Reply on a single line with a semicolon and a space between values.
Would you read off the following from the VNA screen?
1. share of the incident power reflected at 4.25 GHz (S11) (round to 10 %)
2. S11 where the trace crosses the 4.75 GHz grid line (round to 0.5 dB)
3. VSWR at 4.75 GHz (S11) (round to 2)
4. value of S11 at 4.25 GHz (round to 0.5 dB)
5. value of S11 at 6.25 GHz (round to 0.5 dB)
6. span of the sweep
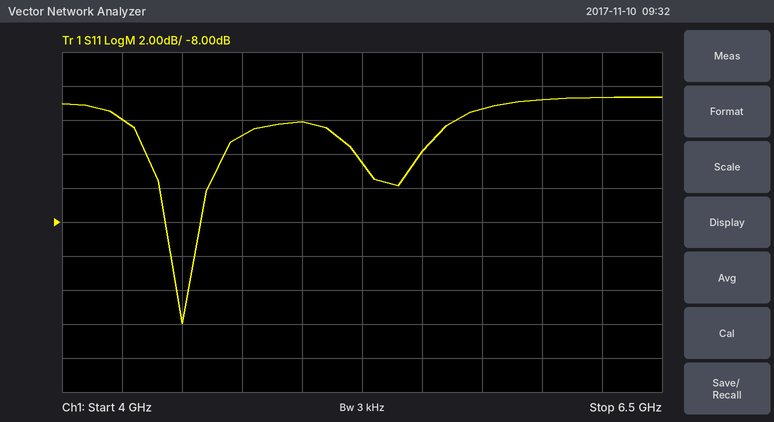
60 %; -3.0 dB; 6; -2.0 dB; -0.5 dB; 2.5 GHz
